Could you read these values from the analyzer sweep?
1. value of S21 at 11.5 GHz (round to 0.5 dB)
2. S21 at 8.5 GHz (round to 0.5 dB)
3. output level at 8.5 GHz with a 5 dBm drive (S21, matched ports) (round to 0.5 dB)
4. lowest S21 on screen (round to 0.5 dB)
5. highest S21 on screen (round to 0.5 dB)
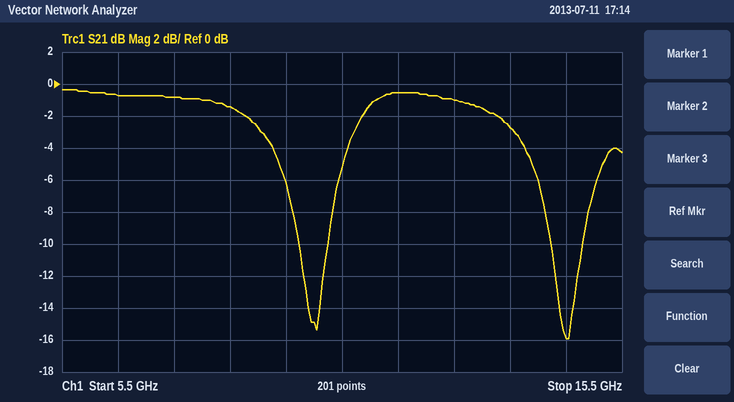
-0.5 dB
-1.5 dB
3.5 dBm
-16.0 dB
-0.5 dB
